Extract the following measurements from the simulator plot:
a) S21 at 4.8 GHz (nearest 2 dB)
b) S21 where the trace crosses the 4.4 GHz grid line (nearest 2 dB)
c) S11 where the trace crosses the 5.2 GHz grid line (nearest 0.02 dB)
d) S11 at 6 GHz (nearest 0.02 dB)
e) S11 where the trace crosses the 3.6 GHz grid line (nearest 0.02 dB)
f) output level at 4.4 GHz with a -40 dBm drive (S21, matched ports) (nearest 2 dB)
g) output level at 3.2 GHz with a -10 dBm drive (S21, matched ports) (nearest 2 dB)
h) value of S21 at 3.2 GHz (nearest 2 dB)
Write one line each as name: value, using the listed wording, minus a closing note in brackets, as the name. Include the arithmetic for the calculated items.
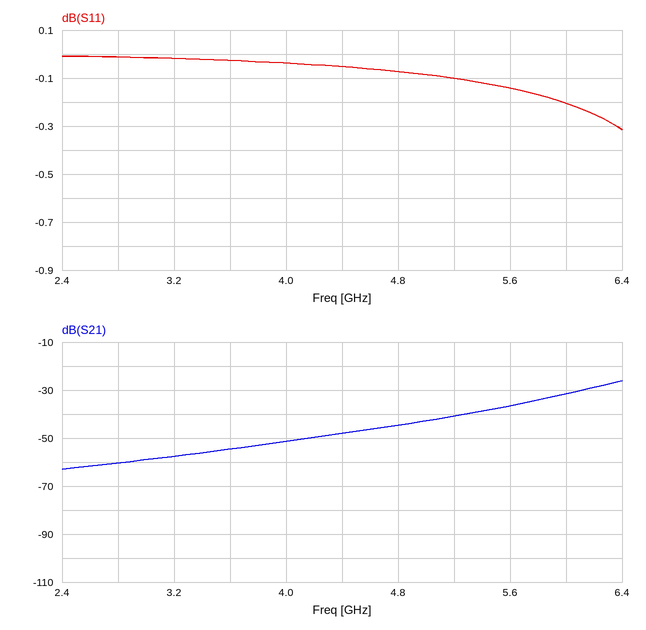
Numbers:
S21 at 4.8 GHz: -44 dB
S21 where the trace crosses the 4.4 GHz grid line: -48 dB
S11 where the trace crosses the 5.2 GHz grid line: -0.10 dB
S11 at 6 GHz: -0.20 dB
S11 where the trace crosses the 3.6 GHz grid line: -0.02 dB
output level at 4.4 GHz with a -40 dBm drive (S21, matched ports): -40 dBm + (-48 dB) = -88 dBm
output level at 3.2 GHz with a -10 dBm drive (S21, matched ports): -10 dBm + (-58 dB) = -68 dBm
value of S21 at 3.2 GHz: -58 dB
